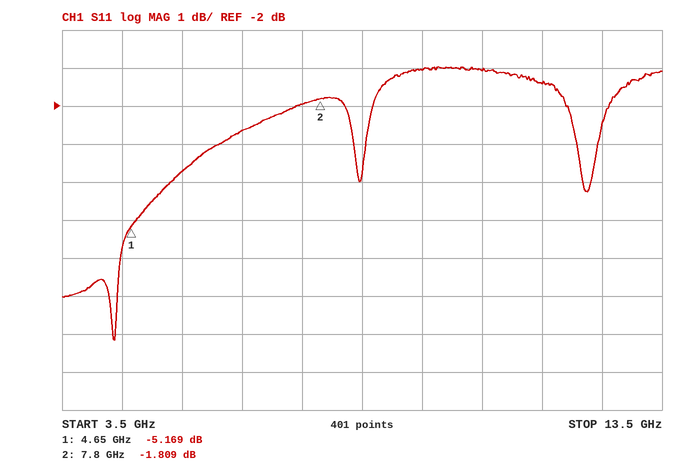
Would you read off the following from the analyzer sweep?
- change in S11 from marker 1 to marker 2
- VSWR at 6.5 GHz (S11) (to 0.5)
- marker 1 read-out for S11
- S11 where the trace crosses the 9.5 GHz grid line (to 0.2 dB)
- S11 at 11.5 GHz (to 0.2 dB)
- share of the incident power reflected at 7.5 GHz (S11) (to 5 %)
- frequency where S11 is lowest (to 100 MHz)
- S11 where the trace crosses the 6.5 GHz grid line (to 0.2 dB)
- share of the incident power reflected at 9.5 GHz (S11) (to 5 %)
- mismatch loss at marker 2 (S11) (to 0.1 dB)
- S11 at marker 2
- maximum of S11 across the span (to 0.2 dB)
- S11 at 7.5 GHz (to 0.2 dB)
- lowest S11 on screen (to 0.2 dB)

3.360 dB
6.5
-5.169 dB
-1.0 dB
-1.4 dB
65 %
4.4 GHz
-2.6 dB
80 %
4.7 dB
-1.809 dB
-1.0 dB
-2.0 dB
-8.2 dB
